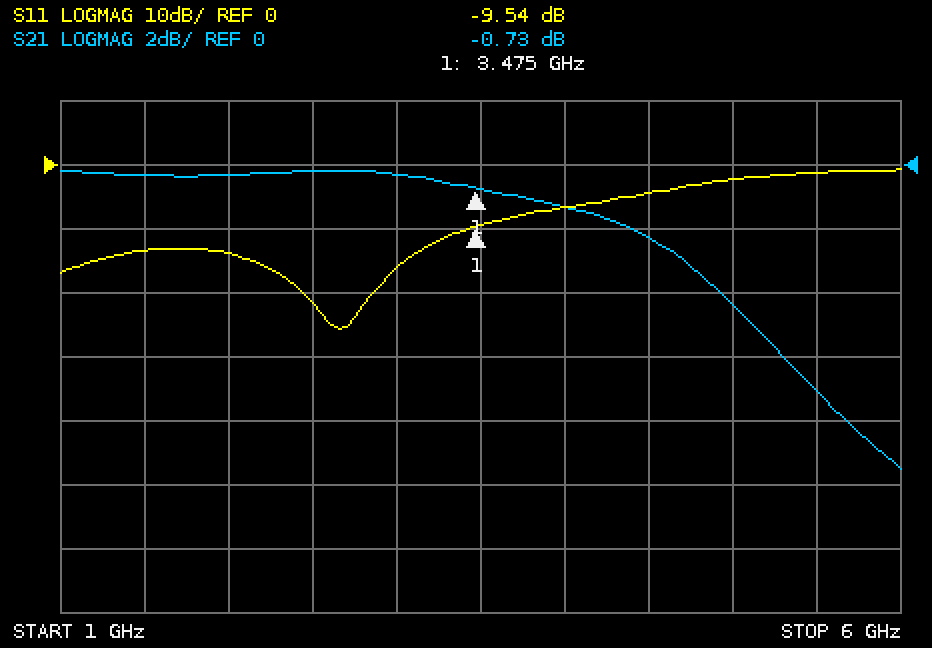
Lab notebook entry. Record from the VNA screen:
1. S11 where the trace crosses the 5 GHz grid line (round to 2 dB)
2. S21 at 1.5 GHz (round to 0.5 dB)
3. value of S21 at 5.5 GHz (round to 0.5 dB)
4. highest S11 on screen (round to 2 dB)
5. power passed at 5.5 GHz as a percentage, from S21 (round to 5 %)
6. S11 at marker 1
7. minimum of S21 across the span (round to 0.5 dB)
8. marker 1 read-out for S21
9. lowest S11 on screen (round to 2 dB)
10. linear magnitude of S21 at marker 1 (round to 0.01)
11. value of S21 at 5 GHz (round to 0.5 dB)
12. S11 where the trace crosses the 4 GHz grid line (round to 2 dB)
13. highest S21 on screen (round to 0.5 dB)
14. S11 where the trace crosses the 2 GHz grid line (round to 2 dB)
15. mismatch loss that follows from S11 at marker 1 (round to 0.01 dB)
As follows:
-2 dB
-0.5 dB
-7.0 dB
0 dB
20 %
-9.54 dB
-9.5 dB
-0.73 dB
-26 dB
0.92
-4.5 dB
-6 dB
0.0 dB
-14 dB
0.51 dB
